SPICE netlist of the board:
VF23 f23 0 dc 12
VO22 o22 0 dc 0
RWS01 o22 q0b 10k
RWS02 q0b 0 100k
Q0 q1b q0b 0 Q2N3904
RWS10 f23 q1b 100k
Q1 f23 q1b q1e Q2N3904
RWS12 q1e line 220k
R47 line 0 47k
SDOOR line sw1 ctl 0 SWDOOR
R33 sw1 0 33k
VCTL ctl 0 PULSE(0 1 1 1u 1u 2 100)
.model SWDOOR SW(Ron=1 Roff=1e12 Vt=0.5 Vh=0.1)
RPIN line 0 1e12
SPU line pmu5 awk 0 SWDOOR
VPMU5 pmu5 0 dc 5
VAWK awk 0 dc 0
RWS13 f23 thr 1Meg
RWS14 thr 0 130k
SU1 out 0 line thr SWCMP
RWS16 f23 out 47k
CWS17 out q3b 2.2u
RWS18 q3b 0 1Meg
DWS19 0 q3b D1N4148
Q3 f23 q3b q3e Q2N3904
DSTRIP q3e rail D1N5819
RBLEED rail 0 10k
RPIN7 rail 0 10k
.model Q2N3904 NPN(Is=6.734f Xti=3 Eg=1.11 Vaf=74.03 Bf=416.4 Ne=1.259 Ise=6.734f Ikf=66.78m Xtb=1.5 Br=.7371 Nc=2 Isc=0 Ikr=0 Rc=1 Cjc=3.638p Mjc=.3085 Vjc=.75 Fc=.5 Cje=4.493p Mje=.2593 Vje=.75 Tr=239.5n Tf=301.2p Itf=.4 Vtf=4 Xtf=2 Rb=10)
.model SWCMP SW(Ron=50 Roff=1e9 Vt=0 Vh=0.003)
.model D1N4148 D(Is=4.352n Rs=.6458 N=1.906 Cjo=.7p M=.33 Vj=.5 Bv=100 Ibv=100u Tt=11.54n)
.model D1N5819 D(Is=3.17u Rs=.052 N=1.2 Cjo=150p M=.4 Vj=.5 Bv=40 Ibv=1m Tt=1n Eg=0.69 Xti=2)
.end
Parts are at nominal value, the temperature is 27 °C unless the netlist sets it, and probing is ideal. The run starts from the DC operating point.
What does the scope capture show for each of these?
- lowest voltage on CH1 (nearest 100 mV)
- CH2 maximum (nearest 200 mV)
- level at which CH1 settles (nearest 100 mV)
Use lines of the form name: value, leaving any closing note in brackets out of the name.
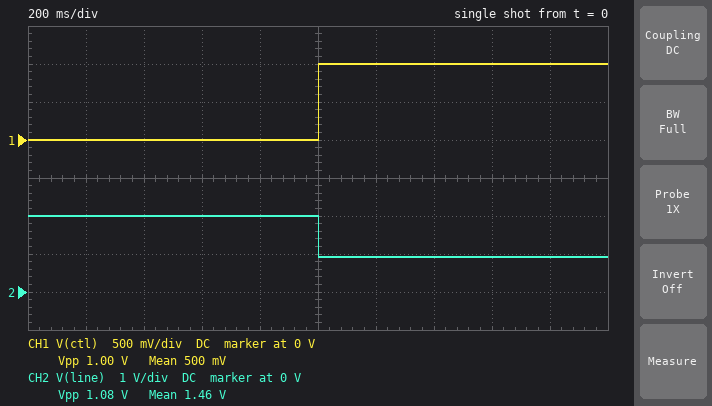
lowest voltage on CH1: 0 V
CH2 maximum: 2.0 V
level at which CH1 settles: 1.0 V
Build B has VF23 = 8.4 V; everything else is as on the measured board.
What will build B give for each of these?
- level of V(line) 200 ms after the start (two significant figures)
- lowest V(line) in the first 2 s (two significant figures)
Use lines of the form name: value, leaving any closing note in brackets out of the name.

level of V(line) 200 ms after the start: 1.4 V
lowest V(line) in the first 2 s: 630 mV
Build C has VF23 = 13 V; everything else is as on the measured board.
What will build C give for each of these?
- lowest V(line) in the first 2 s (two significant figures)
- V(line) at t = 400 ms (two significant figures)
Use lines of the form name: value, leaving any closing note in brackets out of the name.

lowest V(line) in the first 2 s: 1.0 V
V(line) at t = 400 ms: 2.2 V
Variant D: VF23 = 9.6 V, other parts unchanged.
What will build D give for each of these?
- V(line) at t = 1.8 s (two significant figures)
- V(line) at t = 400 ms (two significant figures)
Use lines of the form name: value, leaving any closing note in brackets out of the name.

V(line) at t = 1.8 s: 730 mV
V(line) at t = 400 ms: 1.6 V
